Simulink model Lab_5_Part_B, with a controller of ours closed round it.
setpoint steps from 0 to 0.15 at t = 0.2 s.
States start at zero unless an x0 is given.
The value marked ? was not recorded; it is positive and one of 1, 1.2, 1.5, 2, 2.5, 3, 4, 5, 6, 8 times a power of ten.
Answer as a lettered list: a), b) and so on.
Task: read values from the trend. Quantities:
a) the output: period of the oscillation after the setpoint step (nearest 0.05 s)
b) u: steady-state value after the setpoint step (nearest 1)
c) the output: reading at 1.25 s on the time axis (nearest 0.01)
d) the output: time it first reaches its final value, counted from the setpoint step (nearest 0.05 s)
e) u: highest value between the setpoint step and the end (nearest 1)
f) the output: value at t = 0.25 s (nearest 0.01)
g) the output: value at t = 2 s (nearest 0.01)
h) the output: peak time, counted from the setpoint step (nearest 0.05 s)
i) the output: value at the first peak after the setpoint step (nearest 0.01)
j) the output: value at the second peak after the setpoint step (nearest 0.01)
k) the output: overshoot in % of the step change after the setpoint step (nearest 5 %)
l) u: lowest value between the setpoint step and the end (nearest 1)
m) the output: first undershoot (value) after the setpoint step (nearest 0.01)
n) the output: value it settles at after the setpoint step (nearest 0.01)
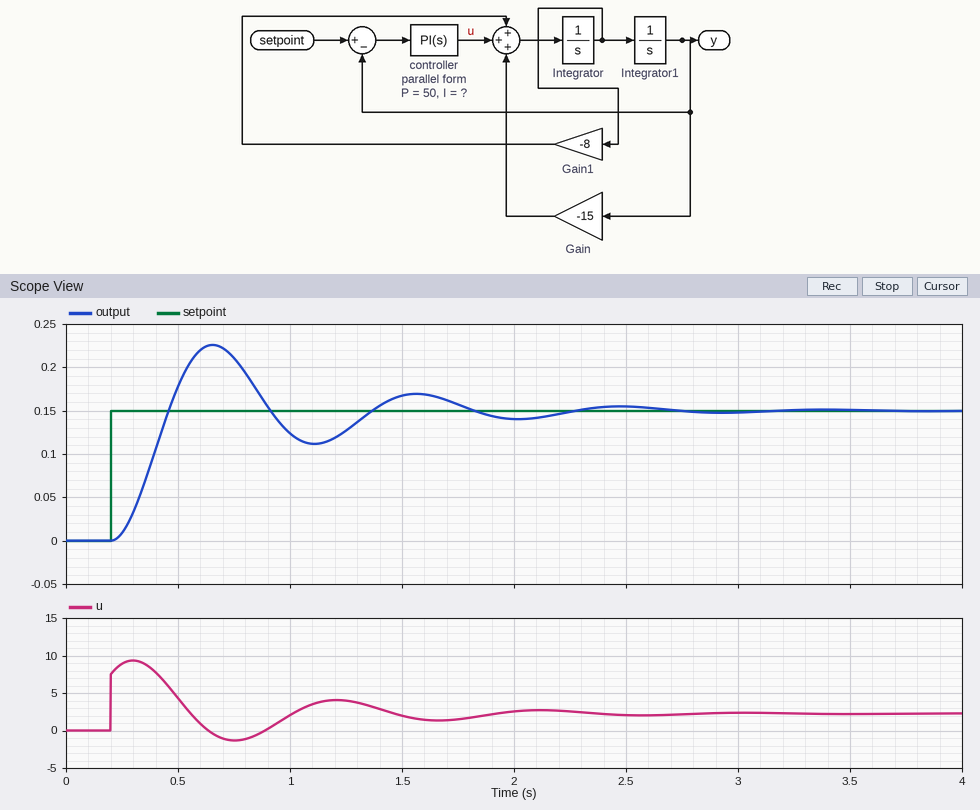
a) 0.90 s
b) 2
c) 0.13
d) 0.25 s
e) 9
f) 0.01
g) 0.14
h) 0.45 s
i) 0.23
j) 0.17
k) 50 %
l) -1
m) 0.11
n) 0.15
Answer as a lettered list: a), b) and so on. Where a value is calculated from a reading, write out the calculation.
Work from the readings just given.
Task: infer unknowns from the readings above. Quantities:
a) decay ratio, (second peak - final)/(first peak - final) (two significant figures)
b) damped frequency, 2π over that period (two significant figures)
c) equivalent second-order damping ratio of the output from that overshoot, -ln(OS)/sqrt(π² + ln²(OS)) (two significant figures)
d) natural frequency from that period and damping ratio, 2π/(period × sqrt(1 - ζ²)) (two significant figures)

a) (0.17 - 0.15) / (0.23 - 0.15) = 0.25
b) 2π / 0.9 = 7.0 rad/s
c) ln(0.5) = -0.693; 0.693 / sqrt(9.870 + 0.480) = 0.22
d) 2π / (0.9 × sqrt(1 - 0.22²)) = 7.2 rad/s
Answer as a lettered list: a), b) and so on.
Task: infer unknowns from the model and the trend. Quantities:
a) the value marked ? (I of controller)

a) 250
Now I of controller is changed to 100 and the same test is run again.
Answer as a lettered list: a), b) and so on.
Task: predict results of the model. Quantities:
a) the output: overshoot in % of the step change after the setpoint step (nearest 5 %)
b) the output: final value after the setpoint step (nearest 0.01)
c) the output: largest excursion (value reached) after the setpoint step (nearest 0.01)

a) 20 %
b) 0.15
c) 0.18
